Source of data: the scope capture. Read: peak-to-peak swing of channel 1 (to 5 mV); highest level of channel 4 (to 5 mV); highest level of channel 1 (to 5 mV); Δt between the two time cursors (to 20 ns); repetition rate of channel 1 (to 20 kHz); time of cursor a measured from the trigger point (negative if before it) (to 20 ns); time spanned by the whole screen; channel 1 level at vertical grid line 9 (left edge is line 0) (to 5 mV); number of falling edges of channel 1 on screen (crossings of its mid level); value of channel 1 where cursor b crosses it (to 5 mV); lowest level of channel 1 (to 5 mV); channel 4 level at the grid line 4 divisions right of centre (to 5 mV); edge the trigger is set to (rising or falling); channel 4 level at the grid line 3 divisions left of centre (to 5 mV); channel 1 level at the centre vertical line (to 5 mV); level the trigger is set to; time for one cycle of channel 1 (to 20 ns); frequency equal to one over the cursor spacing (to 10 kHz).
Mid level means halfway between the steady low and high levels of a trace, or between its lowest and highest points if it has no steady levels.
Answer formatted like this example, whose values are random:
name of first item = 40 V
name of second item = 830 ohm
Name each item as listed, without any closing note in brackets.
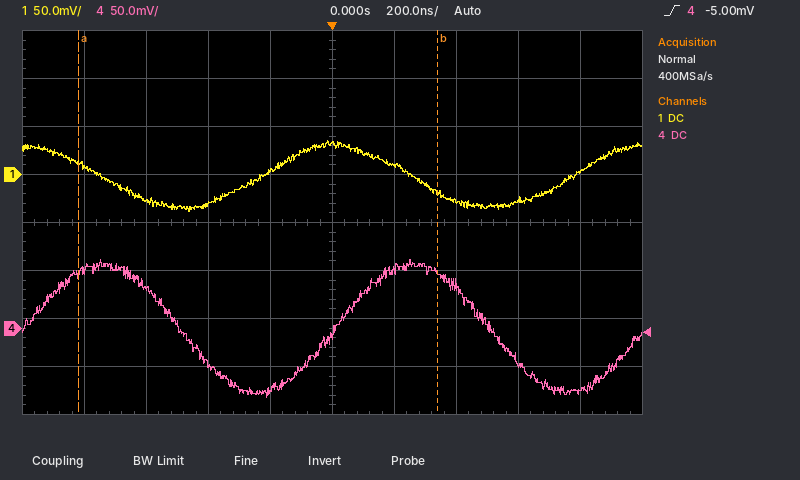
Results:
peak-to-peak swing of channel 1 = 75 mV
highest level of channel 4 = 70 mV
highest level of channel 1 = 35 mV
Δt between the two time cursors = 1.16 µs
repetition rate of channel 1 = 1.00 MHz
time of cursor a measured from the trigger point (negative if before it) = -820 ns
time spanned by the whole screen = 2 µs
channel 1 level at vertical grid line 9 (left edge is line 0) = 5 mV
number of falling edges of channel 1 on screen = 2
value of channel 1 where cursor b crosses it = -20 mV
lowest level of channel 1 = -40 mV
channel 4 level at the grid line 4 divisions right of centre = -65 mV
edge the trigger is set to = rising
channel 4 level at the grid line 3 divisions left of centre = 40 mV
channel 1 level at the centre vertical line = 30 mV
level the trigger is set to = -5.00 mV
time for one cycle of channel 1 = 1.00 µs
frequency equal to one over the cursor spacing = 860 kHz
